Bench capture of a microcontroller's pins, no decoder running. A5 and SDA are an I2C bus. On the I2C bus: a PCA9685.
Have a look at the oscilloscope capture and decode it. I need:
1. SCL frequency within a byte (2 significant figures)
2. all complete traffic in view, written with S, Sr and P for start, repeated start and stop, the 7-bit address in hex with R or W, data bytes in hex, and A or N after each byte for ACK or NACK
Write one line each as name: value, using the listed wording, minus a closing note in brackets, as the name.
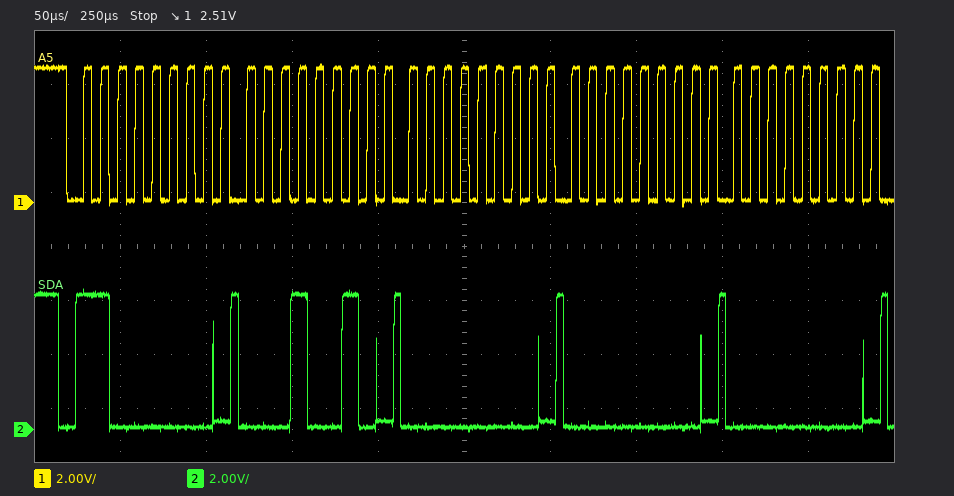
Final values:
SCL frequency within a byte: 100 kHz
all complete traffic in view, written with S, Sr and P for start, repeated start and stop, the 7-bit address in hex with R or W, data bytes in hex, and A or N after each byte for ACK or NACK: S 60W A 12 A 00 A 00 A 00 A
